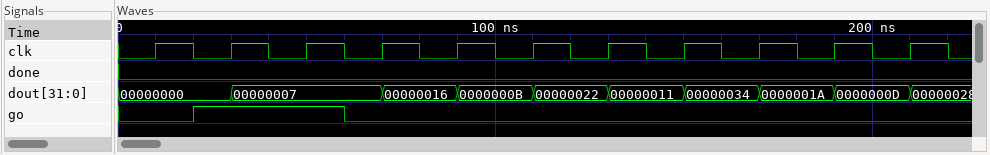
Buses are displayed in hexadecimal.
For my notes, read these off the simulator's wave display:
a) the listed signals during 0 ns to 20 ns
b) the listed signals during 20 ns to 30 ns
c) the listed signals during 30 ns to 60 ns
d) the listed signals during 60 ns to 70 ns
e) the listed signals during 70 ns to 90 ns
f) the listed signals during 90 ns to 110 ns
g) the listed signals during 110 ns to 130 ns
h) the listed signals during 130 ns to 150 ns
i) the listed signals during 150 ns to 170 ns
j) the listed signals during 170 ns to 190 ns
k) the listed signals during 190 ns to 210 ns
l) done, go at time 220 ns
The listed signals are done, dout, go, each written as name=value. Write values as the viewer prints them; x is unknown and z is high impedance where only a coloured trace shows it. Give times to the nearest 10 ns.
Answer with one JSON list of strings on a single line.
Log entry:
["done=0, dout=00000000, go=0", "done=0, dout=00000000, go=1", "done=0, dout=00000007, go=1", "done=0, dout=00000007, go=0", "done=0, dout=00000016, go=0", "done=0, dout=0000000B, go=0", "done=0, dout=00000022, go=0", "done=0, dout=00000011, go=0", "done=0, dout=00000034, go=0", "done=0, dout=0000001A, go=0", "done=0, dout=0000000D, go=0", "done=0, go=0"]
